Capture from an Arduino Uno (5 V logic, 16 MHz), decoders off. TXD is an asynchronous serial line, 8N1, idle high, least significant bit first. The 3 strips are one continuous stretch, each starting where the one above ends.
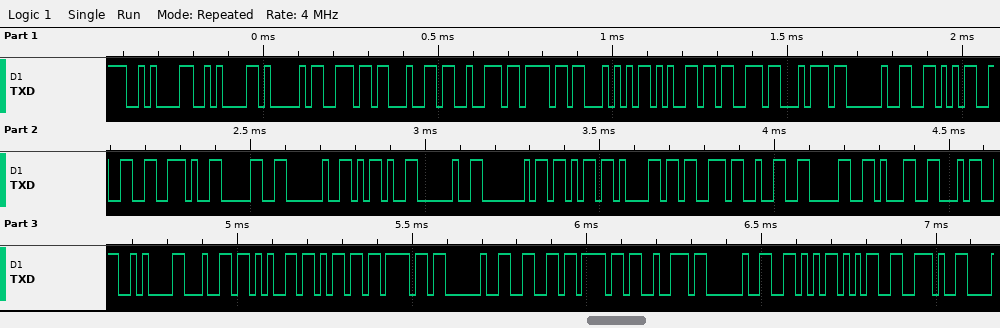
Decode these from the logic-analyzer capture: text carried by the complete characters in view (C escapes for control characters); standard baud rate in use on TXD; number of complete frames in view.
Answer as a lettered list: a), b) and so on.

a) "\n\nAndroTest V2.0 - @kas2014\ndemo for V5."
b) 57600 baud
c) 40
